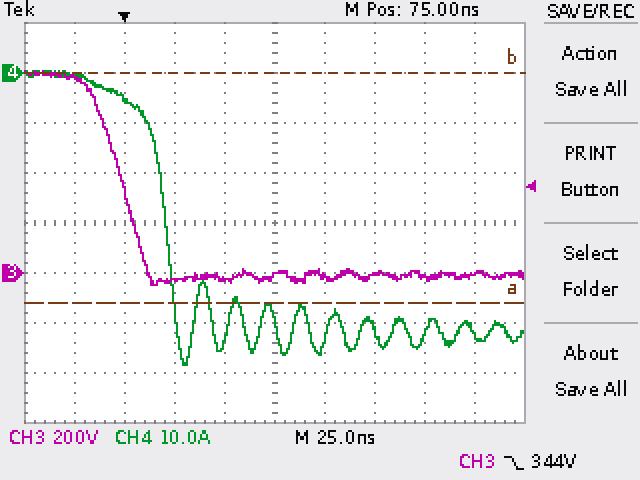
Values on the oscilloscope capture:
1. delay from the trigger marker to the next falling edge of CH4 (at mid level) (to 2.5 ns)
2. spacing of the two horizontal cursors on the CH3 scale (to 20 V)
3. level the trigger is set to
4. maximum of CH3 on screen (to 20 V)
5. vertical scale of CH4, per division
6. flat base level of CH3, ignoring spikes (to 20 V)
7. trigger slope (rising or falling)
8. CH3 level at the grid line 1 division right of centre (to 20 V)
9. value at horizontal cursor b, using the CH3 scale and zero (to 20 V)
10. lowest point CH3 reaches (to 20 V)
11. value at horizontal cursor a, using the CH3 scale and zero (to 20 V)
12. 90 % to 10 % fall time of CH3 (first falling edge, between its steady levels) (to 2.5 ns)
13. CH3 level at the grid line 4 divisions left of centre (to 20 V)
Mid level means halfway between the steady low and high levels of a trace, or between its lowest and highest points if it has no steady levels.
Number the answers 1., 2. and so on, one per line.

1. 20.0 ns
2. 920 V
3. 344 V
4. 800 V
5. 10 A
6. -20 V
7. falling
8. -20 V
9. 800 V
10. -40 V
11. -120 V
12. 25.0 ns
13. 780 V
